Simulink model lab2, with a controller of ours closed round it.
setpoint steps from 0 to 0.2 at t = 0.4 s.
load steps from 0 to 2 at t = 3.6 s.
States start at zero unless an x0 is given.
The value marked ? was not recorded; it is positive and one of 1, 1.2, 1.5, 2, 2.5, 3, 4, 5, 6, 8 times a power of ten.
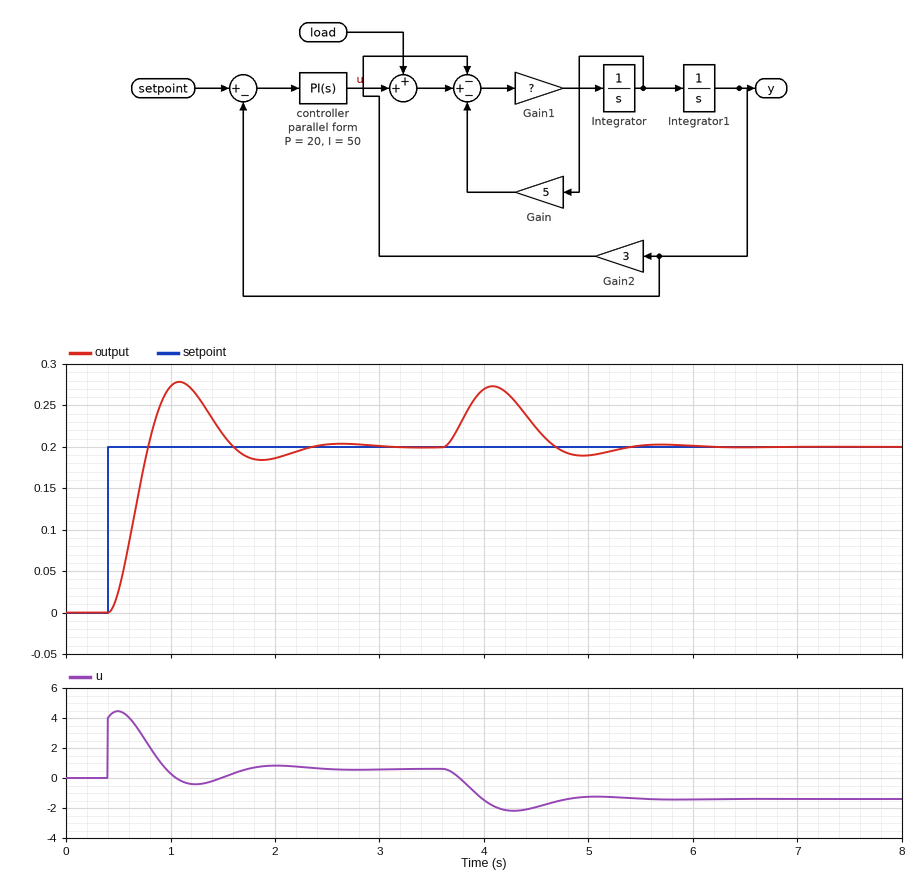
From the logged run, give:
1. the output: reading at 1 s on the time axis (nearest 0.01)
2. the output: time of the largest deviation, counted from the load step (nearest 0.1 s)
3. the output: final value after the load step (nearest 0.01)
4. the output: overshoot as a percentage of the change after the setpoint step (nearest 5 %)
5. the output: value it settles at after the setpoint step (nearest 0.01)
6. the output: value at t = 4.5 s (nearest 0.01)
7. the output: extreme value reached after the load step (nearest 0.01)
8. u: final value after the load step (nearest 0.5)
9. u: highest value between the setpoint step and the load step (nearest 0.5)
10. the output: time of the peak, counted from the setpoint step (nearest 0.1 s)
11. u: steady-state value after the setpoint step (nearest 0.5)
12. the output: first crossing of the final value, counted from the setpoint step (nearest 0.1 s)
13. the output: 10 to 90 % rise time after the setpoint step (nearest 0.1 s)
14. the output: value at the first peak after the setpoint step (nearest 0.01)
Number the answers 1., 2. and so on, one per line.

1. 0.27
2. 0.5 s
3. 0.20
4. 40 %
5. 0.20
6. 0.22
7. 0.27
8. -1.5
9. 4.5
10. 0.7 s
11. 0.5
12. 0.4 s
13. 0.3 s
14. 0.28
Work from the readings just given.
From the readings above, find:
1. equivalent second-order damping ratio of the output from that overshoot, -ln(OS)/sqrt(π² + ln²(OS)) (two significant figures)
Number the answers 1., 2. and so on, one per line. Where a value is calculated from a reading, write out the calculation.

1. ln(0.4) = -0.916; 0.916 / sqrt(9.870 + 0.840) = 0.28
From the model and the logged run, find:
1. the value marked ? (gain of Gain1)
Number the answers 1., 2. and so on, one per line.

1. 1.5
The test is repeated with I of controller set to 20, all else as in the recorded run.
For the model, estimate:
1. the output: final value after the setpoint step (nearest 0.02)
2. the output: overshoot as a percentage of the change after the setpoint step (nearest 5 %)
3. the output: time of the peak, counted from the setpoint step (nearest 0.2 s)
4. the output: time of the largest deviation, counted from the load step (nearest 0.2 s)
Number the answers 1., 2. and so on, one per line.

1. 0.20
2. 15 %
3. 0.8 s
4. 0.6 s
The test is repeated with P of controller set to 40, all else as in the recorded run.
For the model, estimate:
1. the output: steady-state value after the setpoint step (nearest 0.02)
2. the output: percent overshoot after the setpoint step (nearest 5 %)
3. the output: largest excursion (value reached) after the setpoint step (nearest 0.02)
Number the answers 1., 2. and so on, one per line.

1. 0.20
2. 30 %
3. 0.26
